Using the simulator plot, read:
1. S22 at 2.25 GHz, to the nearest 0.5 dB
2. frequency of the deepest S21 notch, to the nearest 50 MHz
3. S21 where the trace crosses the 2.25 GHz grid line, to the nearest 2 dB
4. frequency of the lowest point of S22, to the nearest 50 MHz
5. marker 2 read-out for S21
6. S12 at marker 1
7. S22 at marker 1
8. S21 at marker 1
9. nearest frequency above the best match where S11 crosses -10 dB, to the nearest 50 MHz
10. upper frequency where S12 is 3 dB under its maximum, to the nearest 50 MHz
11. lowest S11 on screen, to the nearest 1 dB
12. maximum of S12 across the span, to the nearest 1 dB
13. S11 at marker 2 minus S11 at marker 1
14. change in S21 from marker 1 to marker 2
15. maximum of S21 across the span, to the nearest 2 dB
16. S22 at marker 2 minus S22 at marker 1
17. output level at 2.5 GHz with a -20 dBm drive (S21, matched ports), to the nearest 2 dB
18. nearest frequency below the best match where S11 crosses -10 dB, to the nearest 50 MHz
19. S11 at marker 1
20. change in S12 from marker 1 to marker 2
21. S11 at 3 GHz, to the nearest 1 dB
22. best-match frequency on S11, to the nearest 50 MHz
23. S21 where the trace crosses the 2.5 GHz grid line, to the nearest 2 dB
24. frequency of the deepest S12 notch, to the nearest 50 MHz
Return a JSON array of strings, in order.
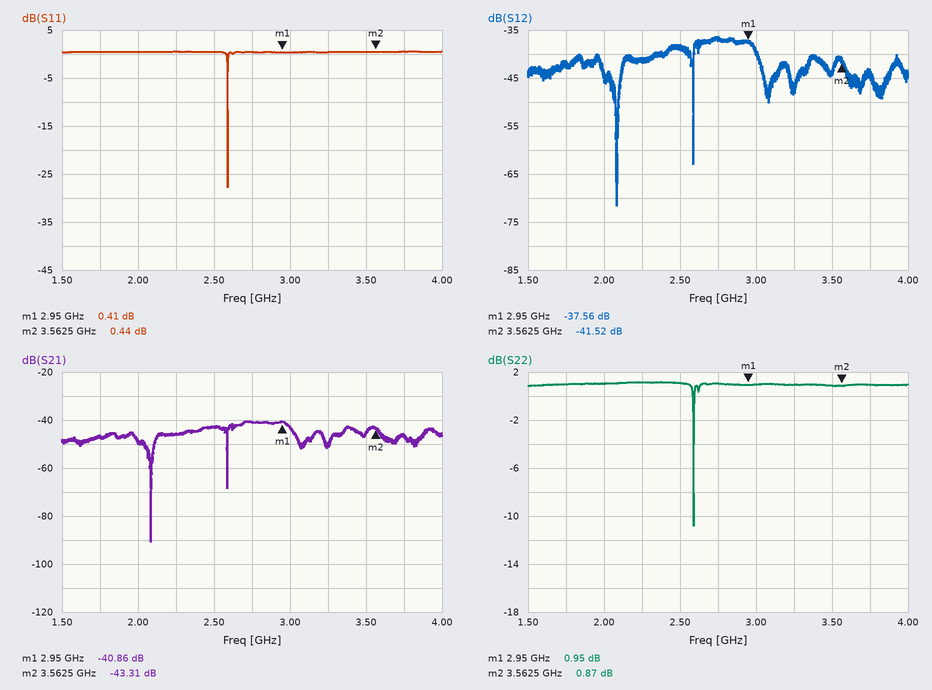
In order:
["1.0 dB", "2.10 GHz", "-46 dB", "2.60 GHz", "-43.31 dB", "-37.56 dB", "0.95 dB", "-40.86 dB", "2.60 GHz", "3.00 GHz", "-28 dB", "-36 dB", "0.03 dB", "-2.45 dB", "-40 dB", "-0.08 dB", "-62 dBm", "2.60 GHz", "0.41 dB", "-3.96 dB", "0 dB", "2.60 GHz", "-42 dB", "2.10 GHz"]
